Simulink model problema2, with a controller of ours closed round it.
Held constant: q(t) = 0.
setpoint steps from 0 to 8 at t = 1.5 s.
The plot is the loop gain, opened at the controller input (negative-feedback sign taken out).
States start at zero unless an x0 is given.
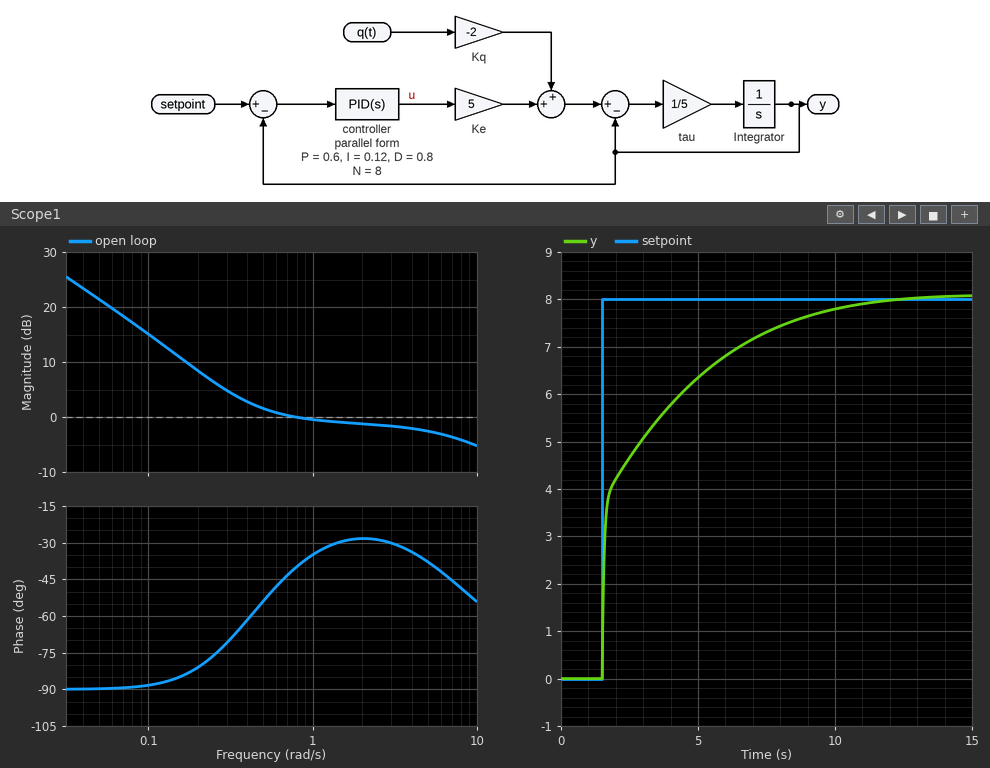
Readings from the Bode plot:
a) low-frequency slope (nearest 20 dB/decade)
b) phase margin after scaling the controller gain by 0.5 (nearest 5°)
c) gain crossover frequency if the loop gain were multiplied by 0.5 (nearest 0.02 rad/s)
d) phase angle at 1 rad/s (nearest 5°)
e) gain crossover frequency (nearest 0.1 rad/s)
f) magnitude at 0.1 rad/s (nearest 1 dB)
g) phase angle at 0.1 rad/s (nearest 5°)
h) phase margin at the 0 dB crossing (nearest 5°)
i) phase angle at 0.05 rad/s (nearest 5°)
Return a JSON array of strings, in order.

["-20 dB/decade", "105°", "0.26 rad/s", "-35°", "0.8 rad/s", "15 dB", "-90°", "140°", "-90°"]
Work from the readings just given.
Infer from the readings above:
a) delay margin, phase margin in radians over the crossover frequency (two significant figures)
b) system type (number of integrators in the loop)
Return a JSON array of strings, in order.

["3.1 s", "1"]
